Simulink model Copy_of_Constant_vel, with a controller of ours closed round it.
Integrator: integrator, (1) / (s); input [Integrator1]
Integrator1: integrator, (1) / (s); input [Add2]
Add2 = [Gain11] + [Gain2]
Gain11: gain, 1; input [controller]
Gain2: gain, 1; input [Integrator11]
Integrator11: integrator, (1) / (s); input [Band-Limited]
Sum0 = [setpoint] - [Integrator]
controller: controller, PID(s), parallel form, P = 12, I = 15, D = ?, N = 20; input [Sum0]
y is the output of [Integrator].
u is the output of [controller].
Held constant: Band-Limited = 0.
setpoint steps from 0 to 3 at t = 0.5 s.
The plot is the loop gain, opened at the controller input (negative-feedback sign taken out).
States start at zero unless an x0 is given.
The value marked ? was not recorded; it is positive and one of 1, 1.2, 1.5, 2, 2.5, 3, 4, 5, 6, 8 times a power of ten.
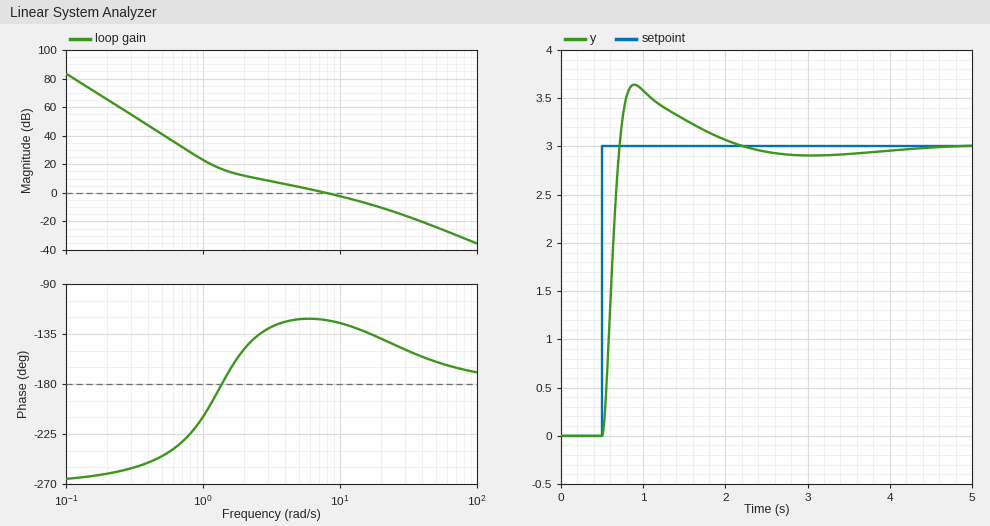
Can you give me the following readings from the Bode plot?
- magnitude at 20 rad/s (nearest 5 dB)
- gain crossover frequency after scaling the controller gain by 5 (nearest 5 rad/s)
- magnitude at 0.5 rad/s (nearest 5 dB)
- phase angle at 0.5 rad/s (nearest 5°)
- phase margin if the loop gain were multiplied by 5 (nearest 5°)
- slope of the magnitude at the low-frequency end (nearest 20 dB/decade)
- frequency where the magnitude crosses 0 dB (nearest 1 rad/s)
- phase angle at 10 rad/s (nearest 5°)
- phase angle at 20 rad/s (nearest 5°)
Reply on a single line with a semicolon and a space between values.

-10 dB; 25 rad/s; 40 dB; -245°; 35°; -60 dB/decade; 8 rad/s; -125°; -140°
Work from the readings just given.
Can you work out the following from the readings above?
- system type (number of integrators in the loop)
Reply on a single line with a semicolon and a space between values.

3
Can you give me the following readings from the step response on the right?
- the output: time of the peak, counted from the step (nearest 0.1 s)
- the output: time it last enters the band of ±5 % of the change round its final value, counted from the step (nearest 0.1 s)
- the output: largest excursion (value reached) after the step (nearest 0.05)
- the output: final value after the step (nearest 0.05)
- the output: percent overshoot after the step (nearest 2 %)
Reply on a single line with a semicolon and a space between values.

0.4 s; 1.3 s; 3.65; 3.00; 22 %
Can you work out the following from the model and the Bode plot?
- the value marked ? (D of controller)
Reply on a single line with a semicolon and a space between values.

8
